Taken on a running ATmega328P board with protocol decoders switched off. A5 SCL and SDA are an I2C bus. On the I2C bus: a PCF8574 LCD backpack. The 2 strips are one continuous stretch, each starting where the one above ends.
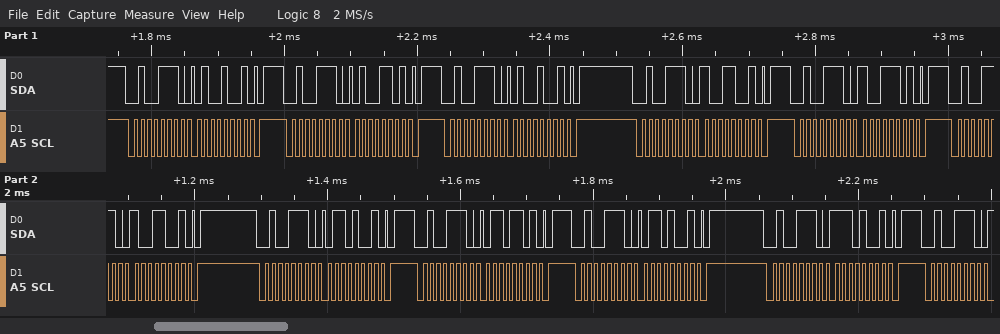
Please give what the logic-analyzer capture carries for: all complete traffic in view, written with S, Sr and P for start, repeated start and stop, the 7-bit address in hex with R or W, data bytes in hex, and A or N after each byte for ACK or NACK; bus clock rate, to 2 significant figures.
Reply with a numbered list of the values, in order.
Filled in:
1. S 27W A 49 A P S 27W A 4D A P S 27W A 49 A P S 27W A 99 A P S 27W A 9D A P S 27W A 99 A P S 27W A 69 A P S 27W A 6D A P S 27W A 69 A P S 27W A E9 A P S 27W A
2. 100 kHz
